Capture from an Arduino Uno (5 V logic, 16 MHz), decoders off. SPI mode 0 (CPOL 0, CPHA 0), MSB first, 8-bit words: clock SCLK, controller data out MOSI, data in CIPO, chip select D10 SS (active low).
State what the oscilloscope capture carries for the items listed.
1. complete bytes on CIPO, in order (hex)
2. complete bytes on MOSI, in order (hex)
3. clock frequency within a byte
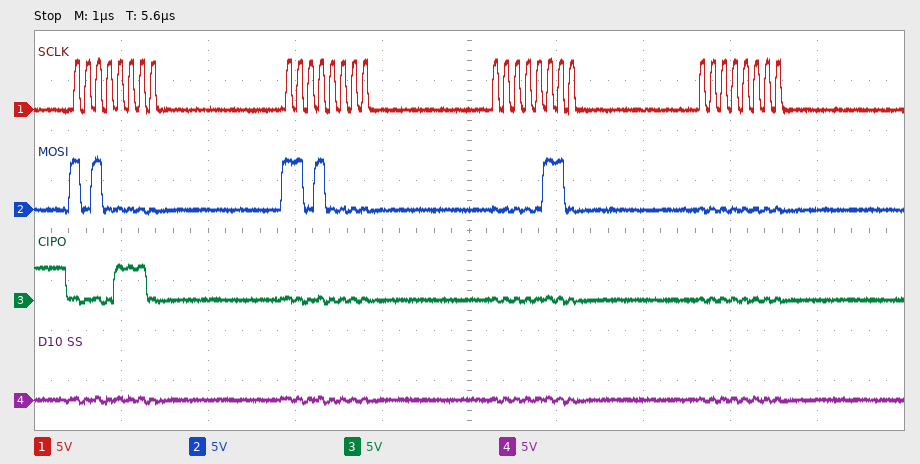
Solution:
0E 00 00 00
A0 D0 06 00
8 MHz
